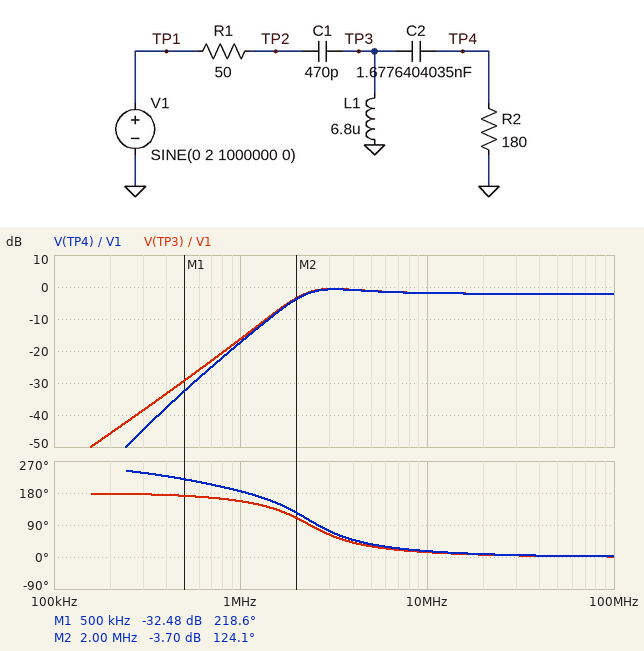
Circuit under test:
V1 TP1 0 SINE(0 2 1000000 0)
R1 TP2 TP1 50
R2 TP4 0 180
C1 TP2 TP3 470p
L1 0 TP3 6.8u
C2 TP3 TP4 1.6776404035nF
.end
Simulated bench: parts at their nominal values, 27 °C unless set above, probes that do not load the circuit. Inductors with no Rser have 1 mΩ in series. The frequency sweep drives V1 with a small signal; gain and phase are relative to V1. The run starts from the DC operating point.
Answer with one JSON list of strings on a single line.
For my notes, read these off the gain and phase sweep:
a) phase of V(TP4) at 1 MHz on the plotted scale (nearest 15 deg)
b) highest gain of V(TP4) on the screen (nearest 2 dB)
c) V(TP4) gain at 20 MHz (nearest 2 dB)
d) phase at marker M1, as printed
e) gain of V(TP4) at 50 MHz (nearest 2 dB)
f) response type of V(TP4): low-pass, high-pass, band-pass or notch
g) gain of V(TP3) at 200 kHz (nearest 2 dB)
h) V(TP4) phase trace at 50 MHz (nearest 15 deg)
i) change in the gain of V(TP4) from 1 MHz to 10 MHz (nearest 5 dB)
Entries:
["180 deg", "0 dB", "-2 dB", "218.6 deg", "-2 dB", "high-pass", "-46 dB", "0 deg", "15 dB"]
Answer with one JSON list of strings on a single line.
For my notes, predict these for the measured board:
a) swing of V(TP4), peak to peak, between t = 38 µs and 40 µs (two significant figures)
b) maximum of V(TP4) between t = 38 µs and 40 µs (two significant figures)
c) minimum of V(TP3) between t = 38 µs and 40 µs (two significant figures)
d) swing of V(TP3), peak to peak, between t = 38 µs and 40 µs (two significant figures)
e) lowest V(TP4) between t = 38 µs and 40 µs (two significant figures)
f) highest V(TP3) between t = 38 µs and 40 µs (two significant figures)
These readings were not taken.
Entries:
["550 mV", "270 mV", "-310 mV", "620 mV", "-270 mV", "310 mV"]
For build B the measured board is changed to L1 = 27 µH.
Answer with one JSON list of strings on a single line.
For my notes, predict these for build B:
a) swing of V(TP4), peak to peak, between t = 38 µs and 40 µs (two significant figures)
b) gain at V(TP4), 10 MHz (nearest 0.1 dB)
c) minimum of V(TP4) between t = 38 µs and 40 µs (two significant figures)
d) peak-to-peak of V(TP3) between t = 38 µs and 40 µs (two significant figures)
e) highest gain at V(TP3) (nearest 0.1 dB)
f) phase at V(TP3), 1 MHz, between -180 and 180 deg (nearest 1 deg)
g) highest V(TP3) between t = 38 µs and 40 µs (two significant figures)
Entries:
["2.1 V", "-2.2 dB", "-1.1 V", "2.4 V", "-2.1 dB", "90 deg", "1.2 V"]
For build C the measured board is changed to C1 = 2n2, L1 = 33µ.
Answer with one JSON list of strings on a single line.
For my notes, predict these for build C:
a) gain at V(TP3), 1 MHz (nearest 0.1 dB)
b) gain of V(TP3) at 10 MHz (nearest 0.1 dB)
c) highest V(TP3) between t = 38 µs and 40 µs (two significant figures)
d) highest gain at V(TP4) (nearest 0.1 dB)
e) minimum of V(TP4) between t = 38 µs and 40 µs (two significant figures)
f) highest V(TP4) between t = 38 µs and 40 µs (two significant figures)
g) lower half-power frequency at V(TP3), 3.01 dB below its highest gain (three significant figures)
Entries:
["-1.0 dB", "-2.1 dB", "1.8 V", "-0.5 dB", "-1.6 V", "1.6 V", "398 kHz"]
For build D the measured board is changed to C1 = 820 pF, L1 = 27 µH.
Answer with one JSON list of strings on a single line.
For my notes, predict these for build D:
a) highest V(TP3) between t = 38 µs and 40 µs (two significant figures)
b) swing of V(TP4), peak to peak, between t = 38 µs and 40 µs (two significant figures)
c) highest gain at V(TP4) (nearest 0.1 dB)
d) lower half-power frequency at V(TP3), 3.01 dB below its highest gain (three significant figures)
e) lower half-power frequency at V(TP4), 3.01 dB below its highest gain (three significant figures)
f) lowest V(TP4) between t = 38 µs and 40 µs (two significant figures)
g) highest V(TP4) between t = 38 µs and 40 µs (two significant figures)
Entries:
["1.7 V", "3.1 V", "-2.1 dB", "627 kHz", "672 kHz", "-1.5 V", "1.5 V"]
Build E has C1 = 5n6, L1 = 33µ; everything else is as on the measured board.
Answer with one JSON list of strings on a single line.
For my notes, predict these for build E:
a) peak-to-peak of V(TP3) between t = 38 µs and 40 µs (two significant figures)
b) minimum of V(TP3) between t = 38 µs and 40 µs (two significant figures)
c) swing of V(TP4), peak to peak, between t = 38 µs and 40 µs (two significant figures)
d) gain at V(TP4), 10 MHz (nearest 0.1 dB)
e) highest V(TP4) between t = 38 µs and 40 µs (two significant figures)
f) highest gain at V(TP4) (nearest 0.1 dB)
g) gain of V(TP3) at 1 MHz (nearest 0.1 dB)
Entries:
["3.4 V", "-1.7 V", "3.0 V", "-2.1 dB", "1.5 V", "-1.9 dB", "-1.4 dB"]
